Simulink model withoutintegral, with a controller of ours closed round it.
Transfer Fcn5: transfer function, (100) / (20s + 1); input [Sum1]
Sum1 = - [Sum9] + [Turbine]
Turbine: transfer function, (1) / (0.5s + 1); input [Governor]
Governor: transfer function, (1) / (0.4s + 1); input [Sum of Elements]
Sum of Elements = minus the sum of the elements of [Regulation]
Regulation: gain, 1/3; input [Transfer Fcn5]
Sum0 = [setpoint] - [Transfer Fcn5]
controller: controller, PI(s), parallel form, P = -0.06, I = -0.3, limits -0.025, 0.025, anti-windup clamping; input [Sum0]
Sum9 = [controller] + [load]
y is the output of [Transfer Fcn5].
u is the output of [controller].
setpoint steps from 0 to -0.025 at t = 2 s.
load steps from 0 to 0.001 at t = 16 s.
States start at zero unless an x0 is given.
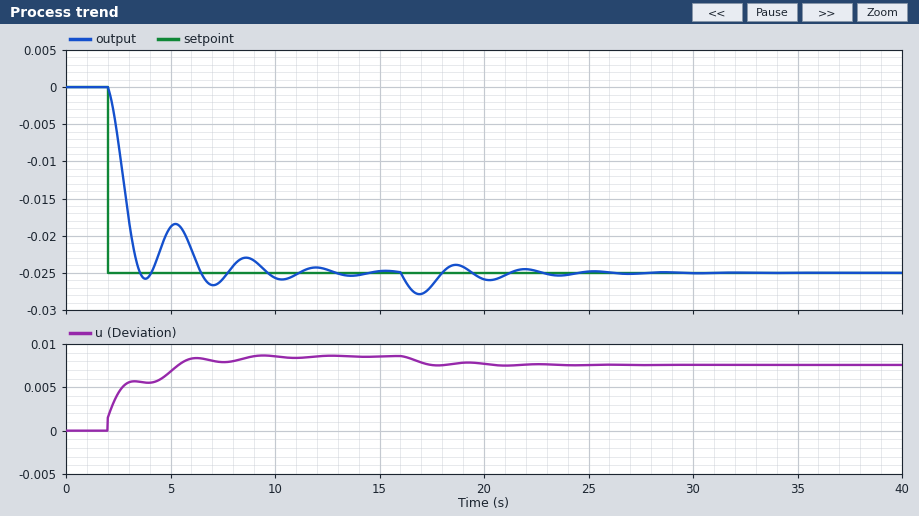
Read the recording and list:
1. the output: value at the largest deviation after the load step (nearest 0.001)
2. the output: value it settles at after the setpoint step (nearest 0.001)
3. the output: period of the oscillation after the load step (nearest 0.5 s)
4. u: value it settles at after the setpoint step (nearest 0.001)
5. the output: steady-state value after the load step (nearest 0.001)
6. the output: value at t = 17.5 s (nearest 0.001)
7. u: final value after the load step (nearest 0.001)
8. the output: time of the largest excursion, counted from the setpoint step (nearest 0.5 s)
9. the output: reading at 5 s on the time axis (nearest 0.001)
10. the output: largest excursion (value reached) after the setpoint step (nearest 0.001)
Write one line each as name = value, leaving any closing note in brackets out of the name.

the output: value at the largest deviation after the load step = -0.028
the output: value it settles at after the setpoint step = -0.025
the output: period of the oscillation after the load step = 3.5 s
u: value it settles at after the setpoint step = 0.009
the output: steady-state value after the load step = -0.025
the output: value at t = 17.5 s = -0.027
u: final value after the load step = 0.008
the output: time of the largest excursion, counted from the setpoint step = 5.0 s
the output: reading at 5 s on the time axis = -0.019
the output: largest excursion (value reached) after the setpoint step = -0.027
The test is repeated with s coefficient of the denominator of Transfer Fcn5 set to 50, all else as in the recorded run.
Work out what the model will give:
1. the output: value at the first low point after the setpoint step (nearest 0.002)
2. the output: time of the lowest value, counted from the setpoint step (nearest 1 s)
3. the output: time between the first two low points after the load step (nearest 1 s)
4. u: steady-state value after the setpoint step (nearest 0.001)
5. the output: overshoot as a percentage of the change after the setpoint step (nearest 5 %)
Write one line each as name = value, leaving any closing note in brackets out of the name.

the output: value at the first low point after the setpoint step = -0.028
the output: time of the lowest value, counted from the setpoint step = 3 s
the output: time between the first two low points after the load step = 6 s
u: steady-state value after the setpoint step = 0.009
the output: overshoot as a percentage of the change after the setpoint step = 15 %
